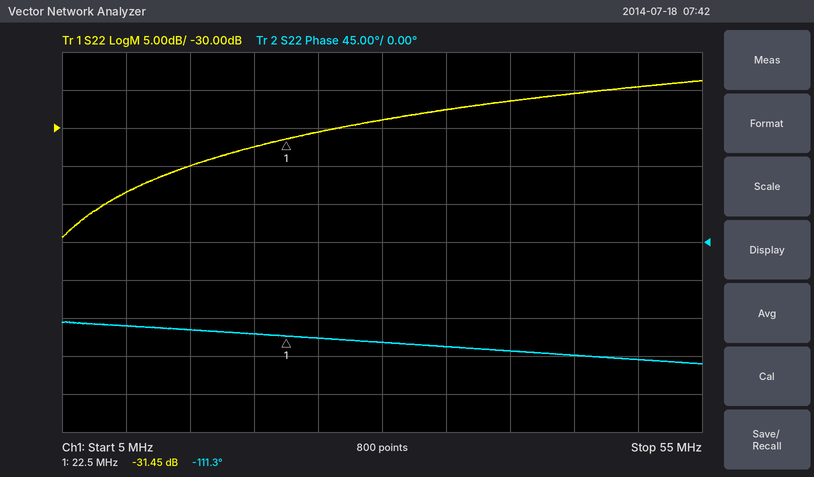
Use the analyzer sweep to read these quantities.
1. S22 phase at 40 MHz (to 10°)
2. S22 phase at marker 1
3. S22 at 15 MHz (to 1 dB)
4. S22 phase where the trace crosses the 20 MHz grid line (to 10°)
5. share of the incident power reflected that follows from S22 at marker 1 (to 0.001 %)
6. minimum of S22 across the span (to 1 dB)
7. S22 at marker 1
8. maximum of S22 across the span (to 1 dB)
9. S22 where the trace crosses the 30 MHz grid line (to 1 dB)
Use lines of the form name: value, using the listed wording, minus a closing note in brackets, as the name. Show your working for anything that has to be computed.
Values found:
S22 phase at 40 MHz: -130°
S22 phase at marker 1: -111.3°
S22 at 15 MHz: -35 dB
S22 phase where the trace crosses the 20 MHz grid line: -110°
share of the incident power reflected that follows from S22 at marker 1: 10^(-31.45/10) ≈ 0.072 %
minimum of S22 across the span: -44 dB
S22 at marker 1: -31.45 dB
maximum of S22 across the span: -24 dB
S22 where the trace crosses the 30 MHz grid line: -29 dB
